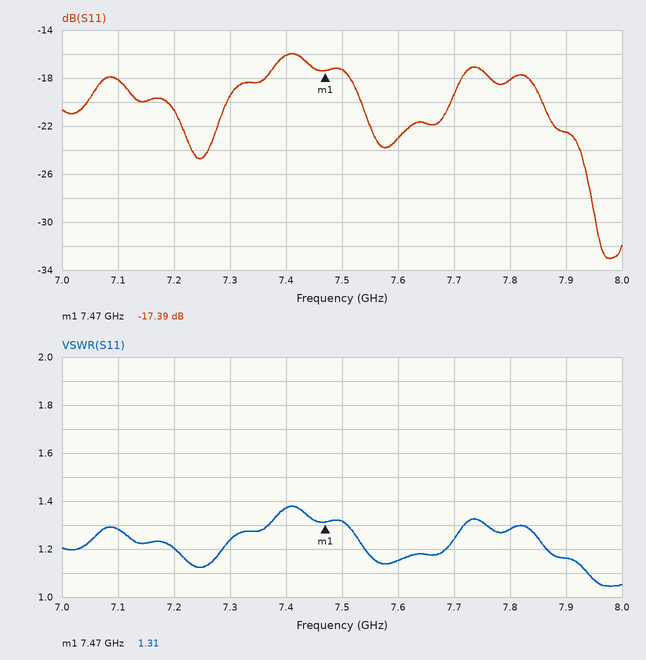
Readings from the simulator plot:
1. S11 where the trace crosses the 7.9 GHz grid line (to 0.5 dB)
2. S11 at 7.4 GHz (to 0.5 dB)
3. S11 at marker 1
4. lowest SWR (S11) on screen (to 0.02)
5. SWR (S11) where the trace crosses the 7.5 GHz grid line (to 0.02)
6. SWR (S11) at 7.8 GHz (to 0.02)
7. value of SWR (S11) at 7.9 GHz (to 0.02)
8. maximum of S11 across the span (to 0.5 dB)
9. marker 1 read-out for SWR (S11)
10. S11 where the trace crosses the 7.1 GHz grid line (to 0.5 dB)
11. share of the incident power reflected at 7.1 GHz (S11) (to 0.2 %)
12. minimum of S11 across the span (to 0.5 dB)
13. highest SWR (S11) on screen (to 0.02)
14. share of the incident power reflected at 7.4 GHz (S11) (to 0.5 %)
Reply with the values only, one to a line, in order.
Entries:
-22.5 dB
-16.0 dB
-17.39 dB
1.04
1.32
1.28
1.16
-16.0 dB
1.31
-18.0 dB
1.6 %
-33.0 dB
1.38
2.5 %
